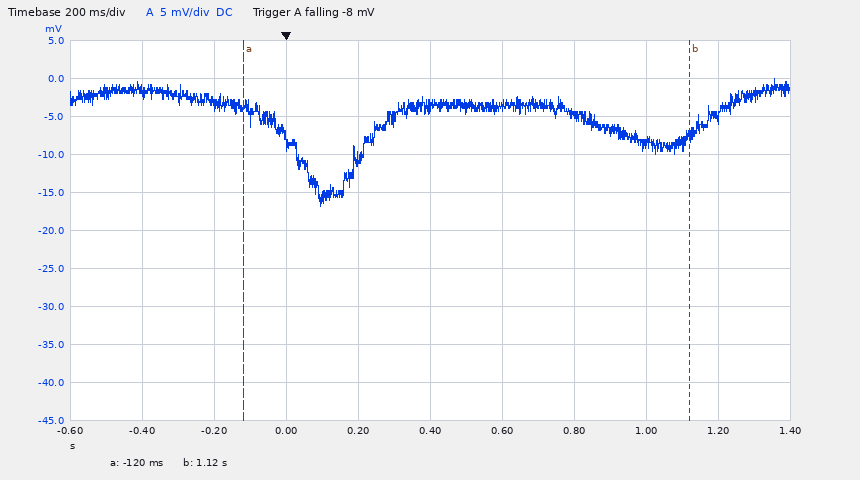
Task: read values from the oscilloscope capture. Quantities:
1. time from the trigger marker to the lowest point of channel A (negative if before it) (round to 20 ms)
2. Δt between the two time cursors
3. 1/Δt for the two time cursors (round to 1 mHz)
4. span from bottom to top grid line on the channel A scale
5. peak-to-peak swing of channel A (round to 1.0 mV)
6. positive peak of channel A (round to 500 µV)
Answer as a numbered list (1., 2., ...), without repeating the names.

1. +100 ms
2. 1.24 s
3. 806 mHz
4. 50 mV
5. 17.0 mV
6. 0.0 mV
